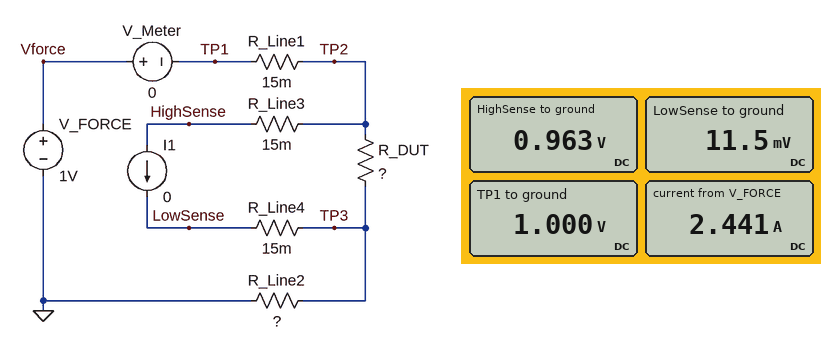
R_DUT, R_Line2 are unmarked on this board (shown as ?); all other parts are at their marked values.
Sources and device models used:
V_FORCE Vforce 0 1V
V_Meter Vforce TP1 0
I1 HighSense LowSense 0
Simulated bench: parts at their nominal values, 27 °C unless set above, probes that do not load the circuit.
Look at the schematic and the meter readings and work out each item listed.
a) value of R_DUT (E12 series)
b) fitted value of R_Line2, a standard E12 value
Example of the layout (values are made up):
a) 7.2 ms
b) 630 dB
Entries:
a) 0.39 Ω
b) 4.7 mΩ
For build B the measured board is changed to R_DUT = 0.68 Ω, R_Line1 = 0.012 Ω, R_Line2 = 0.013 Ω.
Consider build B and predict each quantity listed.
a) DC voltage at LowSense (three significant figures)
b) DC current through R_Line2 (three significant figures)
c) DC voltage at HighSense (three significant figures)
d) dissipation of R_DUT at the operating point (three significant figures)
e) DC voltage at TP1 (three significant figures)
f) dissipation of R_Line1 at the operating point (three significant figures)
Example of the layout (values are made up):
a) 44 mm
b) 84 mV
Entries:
a) 18.4 mV
b) 1.42 A
c) 983 mV
d) 1.37 W
e) 1.00 V
f) 24.1 mW
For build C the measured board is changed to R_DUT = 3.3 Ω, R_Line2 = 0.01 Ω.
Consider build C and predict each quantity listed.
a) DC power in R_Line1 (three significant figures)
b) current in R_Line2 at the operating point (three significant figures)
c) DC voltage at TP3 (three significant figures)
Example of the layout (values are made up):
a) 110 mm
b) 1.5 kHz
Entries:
a) 1.36 mW
b) 301 mA
c) 3.01 mV
